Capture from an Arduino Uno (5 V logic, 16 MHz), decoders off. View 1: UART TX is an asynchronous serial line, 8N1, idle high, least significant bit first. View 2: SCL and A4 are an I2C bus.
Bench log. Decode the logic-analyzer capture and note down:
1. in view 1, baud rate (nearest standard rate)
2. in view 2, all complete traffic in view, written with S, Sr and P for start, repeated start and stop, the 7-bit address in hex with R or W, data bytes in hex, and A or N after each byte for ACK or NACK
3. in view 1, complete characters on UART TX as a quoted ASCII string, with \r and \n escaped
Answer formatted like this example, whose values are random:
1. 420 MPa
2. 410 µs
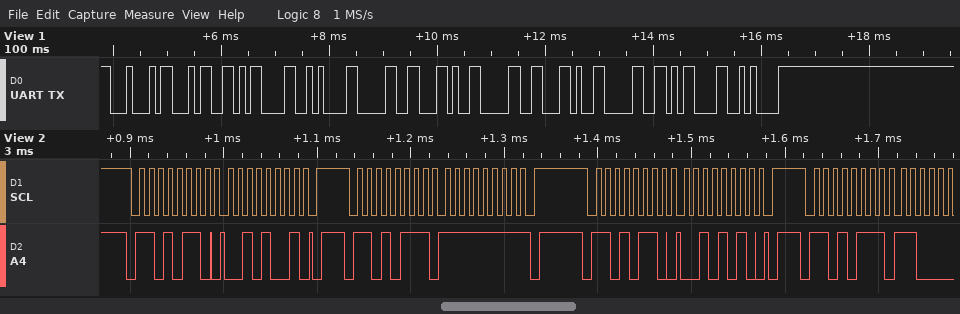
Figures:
1. 9600 baud
2. S 6BW A 29 A P S 6BR A FF N P S 6BW A 2A A P S 6BR A
3. "D4\r\n0,0,0\r\n"
